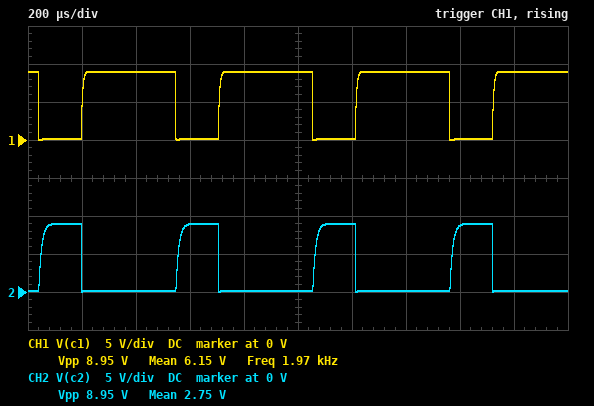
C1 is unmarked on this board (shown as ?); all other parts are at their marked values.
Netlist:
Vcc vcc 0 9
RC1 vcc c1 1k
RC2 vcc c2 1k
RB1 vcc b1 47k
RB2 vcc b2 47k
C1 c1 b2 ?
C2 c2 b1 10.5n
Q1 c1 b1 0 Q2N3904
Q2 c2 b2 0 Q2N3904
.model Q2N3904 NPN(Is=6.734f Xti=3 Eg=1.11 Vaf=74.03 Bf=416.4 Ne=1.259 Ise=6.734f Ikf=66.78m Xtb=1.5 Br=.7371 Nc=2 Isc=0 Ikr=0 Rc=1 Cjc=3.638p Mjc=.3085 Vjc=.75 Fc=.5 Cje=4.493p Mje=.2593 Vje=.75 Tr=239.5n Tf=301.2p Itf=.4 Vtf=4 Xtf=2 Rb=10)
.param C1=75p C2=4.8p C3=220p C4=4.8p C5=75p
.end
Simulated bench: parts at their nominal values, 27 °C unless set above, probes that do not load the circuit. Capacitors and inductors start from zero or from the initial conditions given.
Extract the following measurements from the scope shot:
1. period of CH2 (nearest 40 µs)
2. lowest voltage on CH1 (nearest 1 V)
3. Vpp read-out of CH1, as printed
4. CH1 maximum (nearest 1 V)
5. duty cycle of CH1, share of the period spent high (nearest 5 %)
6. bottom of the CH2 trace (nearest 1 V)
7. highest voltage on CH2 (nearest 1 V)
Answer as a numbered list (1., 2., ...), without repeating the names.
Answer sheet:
1. 520 µs
2. 0 V
3. 8.95 V
4. 9 V
5. 70 %
6. 0 V
7. 9 V
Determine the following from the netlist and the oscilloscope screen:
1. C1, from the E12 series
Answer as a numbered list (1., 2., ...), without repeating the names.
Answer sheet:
1. 4.7 nF
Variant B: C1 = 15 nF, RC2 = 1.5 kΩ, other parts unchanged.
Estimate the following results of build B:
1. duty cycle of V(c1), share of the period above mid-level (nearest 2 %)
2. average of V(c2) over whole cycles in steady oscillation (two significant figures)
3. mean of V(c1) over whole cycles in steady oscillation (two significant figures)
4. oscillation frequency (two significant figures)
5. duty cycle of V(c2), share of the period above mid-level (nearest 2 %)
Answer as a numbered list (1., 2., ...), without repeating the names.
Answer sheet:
1. 40 %
2. 5.2 V
3. 3.6 V
4. 1.2 kHz
5. 58 %
